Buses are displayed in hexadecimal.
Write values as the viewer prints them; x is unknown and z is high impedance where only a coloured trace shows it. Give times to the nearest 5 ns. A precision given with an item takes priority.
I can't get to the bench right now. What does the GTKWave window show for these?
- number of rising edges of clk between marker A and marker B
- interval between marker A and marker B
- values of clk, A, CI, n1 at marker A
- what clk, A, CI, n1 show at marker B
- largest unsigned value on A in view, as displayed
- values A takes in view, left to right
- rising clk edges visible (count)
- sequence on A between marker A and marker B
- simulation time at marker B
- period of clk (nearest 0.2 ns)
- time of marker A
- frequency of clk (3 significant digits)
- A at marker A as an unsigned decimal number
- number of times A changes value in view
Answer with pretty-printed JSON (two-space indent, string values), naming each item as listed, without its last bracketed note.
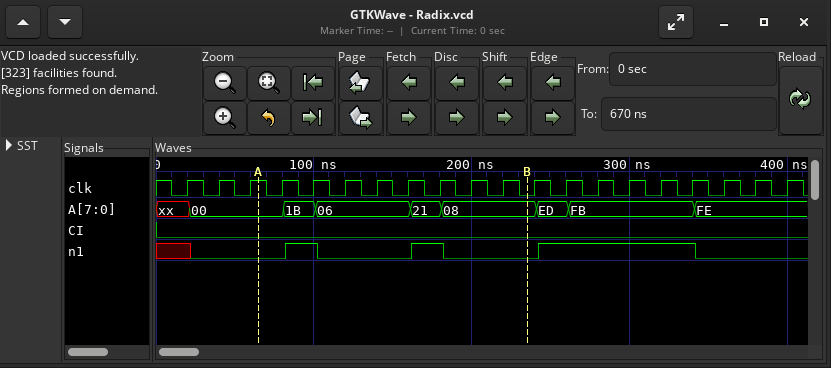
{
  "number of rising edges of clk between marker A and marker B": "8",
  "interval between marker A and marker B": "170 ns",
  "values of clk, A, CI, n1 at marker A": "clk=1, A=00, CI=0, n1=0",
  "what clk, A, CI, n1 show at marker B": "clk=0, A=08, CI=0, n1=0",
  "largest unsigned value on A in view, as displayed": "FE",
  "values A takes in view, left to right": "xx, 00, 1B, 06, 21, 08, ED, FB, FE",
  "rising clk edges visible": "20",
  "sequence on A between marker A and marker B": "00, 1B, 06, 21, 08",
  "simulation time at marker B": "235 ns",
  "period of clk": "20 ns",
  "time of marker A": "65 ns",
  "frequency of clk": "50.0 MHz",
  "A at marker A as an unsigned decimal number": "0",
  "number of times A changes value in view": "8"
}
